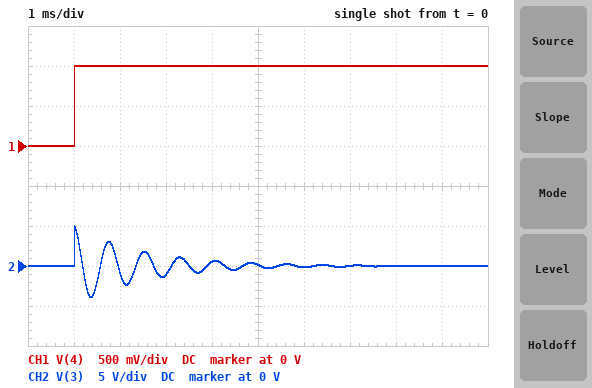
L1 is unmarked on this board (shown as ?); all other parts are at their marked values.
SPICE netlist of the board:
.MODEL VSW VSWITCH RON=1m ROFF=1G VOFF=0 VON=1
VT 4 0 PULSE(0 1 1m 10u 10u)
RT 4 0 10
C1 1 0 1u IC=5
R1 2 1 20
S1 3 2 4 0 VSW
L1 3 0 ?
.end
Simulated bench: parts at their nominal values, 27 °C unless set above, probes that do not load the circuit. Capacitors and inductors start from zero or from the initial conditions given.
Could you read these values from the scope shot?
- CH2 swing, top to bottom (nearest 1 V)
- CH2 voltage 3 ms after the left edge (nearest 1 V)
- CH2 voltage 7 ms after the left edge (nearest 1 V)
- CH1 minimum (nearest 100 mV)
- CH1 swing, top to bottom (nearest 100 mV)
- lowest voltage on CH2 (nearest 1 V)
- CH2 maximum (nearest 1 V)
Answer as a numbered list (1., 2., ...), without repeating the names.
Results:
1. 9 V
2. -1 V
3. 0 V
4. 0 V
5. 1.0 V
6. -4 V
7. 5 V
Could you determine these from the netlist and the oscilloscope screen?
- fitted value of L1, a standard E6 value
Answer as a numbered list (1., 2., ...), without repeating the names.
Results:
1. 15 mH
